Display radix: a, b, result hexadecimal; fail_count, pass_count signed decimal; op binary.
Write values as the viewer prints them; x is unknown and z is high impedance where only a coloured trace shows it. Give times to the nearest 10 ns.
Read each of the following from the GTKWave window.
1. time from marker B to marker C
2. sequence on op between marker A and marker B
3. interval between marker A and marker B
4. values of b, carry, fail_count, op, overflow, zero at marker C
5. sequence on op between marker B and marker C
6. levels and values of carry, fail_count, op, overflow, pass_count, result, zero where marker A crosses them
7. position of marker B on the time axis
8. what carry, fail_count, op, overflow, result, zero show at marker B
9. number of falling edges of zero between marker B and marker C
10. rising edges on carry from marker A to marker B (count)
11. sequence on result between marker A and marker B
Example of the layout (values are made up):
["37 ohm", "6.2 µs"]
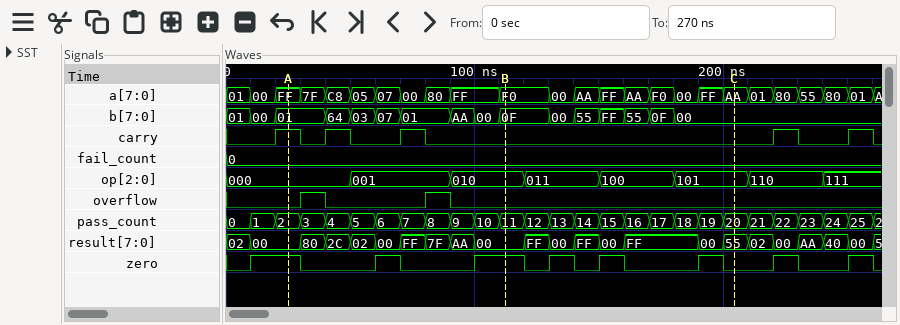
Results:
["90 ns", "000, 001, 010", "90 ns", "b=00, carry=0, fail_count=0, op=101, overflow=0, zero=0", "010, 011, 100, 101", "carry=1, fail_count=0, op=000, overflow=0, pass_count=2, result=00, zero=1", "110 ns", "carry=0, fail_count=0, op=010, overflow=0, result=00, zero=1", "4", "2", "00, 80, 2C, 02, 00, FF, 7F, AA, 00"]
